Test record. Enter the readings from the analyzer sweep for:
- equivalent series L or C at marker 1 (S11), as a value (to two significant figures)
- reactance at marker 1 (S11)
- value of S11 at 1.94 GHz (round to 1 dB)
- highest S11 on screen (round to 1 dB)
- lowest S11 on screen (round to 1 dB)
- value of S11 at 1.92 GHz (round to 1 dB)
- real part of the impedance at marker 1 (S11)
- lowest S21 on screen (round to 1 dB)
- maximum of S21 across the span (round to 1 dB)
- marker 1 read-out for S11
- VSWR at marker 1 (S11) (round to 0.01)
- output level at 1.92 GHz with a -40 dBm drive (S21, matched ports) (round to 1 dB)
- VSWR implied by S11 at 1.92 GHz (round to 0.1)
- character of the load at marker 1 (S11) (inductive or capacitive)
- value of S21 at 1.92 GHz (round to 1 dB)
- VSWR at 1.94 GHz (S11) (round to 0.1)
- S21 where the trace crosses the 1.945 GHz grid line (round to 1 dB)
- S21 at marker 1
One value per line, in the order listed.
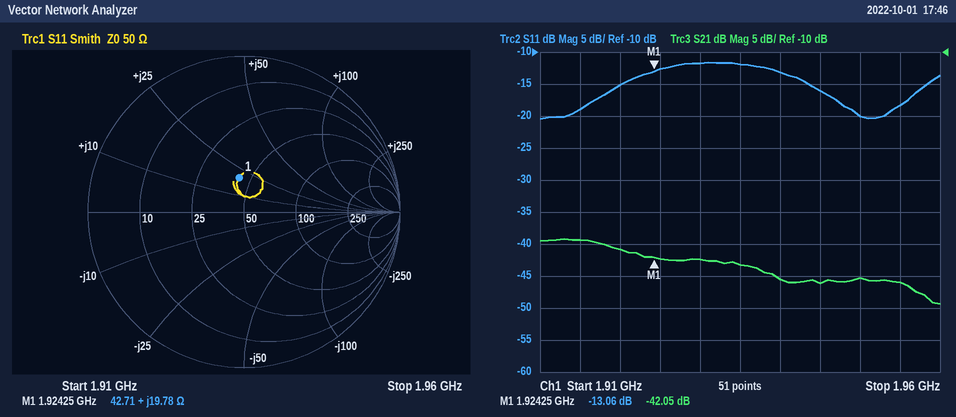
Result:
1.6 nH
+19.78 Ω
-13 dB
-12 dB
-20 dB
-15 dB
42.71 Ω
-49 dB
-39 dB
-13.06 dB
1.57
-81 dBm
1.4
inductive
-41 dB
1.6
-46 dB
-42.05 dB
